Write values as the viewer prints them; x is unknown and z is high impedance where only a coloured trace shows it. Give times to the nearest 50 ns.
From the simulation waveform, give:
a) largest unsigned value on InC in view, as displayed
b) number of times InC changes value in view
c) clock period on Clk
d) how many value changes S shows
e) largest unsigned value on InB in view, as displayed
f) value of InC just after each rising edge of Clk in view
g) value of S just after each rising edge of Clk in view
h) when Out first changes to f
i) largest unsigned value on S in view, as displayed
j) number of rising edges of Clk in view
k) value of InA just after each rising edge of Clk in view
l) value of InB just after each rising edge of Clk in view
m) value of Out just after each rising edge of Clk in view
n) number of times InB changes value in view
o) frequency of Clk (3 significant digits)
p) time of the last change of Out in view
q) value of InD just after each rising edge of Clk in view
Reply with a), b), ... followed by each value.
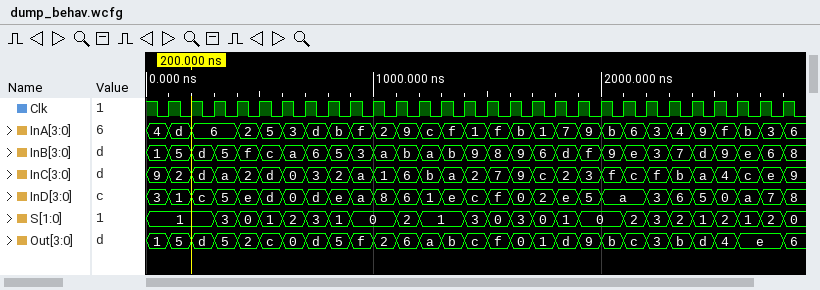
a) f
b) 28
c) 100 ns
d) 23
e) f
f) 2, d, a, 2, d, 0, 3, 2, a, 1, 6, b, a, 2, 7, 9, c, 2, 3, f, c, f, b, a, 4, c, e, 9
g) 1, 1, 3, 0, 1, 2, 3, 1, 0, 0, 2, 1, 1, 3, 0, 3, 0, 1, 0, 0, 2, 3, 2, 1, 2, 1, 2, 0
h) 900 ns
i) 3
j) 28
k) d, 6, 6, 2, 5, 3, d, b, f, 2, 9, c, f, 1, f, b, 1, 7, 9, b, 6, 3, 4, 9, f, b, 3, 6
l) 5, d, 5, f, c, a, 6, 5, 3, a, b, a, b, 9, 8, 9, 6, d, f, 9, e, 3, 7, d, 9, e, 6, 8
m) 5, d, 5, 2, c, 0, d, 5, f, 2, 6, a, b, c, f, 0, 1, d, 9, b, c, 3, b, d, 4, e, e, 6
n) 28
o) 10.0 MHz
p) 2800 ns
q) 1, c, 5, e, d, 0, d, e, a, 8, 6, 1, e, c, f, 0, 2, e, 5, a, a, 3, 6, 5, 0, a, 7, 8
